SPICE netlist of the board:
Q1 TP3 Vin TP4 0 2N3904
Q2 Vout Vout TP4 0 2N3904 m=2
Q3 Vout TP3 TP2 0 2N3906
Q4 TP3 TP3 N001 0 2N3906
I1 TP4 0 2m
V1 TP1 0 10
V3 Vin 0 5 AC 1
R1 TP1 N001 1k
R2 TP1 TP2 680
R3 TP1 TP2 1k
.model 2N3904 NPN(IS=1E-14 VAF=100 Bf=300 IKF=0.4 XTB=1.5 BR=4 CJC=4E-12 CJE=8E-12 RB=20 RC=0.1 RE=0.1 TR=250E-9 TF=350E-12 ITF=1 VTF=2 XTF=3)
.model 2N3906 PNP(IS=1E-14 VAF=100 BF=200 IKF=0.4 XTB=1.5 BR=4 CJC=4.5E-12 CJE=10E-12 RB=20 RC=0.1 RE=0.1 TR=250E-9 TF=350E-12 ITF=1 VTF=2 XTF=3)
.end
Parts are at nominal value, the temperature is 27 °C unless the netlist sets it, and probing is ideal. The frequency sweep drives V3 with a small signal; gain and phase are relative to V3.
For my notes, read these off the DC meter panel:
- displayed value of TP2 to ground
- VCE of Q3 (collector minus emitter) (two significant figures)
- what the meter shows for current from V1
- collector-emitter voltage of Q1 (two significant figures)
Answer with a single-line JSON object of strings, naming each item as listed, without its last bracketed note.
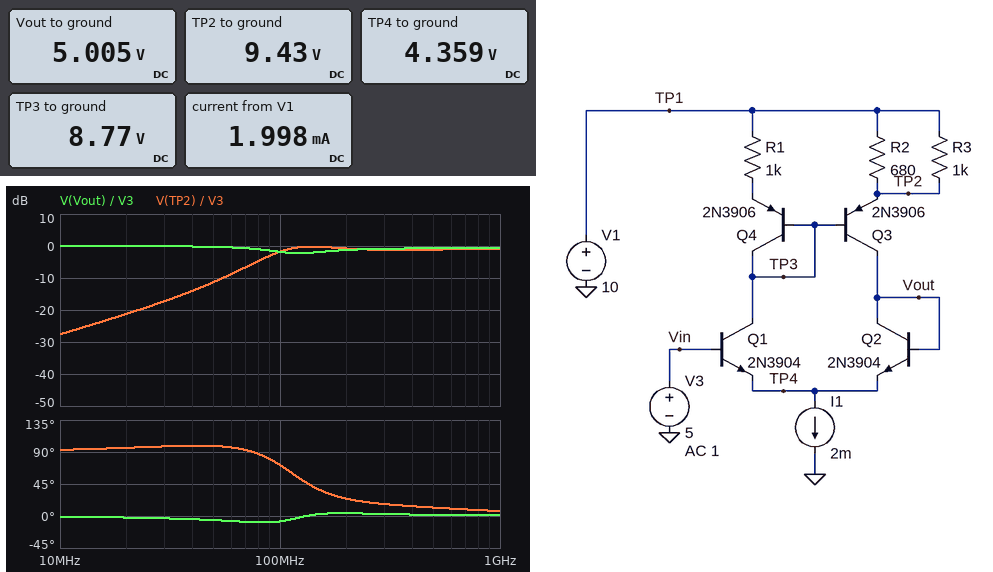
{"displayed value of TP2 to ground": "9.43 V", "VCE of Q3 (collector minus emitter)": "-4.4 V", "what the meter shows for current from V1": "1.998 mA", "collector-emitter voltage of Q1": "4.4 V"}
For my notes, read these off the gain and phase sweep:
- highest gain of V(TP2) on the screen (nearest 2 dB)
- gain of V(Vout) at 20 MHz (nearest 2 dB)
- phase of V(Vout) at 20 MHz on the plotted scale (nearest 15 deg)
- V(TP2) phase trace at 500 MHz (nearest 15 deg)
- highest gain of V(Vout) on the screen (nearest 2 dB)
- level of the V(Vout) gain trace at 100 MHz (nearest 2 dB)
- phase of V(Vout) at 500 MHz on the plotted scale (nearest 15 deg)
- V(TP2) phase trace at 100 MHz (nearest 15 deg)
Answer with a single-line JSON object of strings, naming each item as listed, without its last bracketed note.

{"highest gain of V(TP2) on the screen": "0 dB", "gain of V(Vout) at 20 MHz": "0 dB", "phase of V(Vout) at 20 MHz on the plotted scale": "0 deg", "V(TP2) phase trace at 500 MHz": "15 deg", "highest gain of V(Vout) on the screen": "0 dB", "level of the V(Vout) gain trace at 100 MHz": "-2 dB", "phase of V(Vout) at 500 MHz on the plotted scale": "0 deg", "V(TP2) phase trace at 100 MHz": "75 deg"}
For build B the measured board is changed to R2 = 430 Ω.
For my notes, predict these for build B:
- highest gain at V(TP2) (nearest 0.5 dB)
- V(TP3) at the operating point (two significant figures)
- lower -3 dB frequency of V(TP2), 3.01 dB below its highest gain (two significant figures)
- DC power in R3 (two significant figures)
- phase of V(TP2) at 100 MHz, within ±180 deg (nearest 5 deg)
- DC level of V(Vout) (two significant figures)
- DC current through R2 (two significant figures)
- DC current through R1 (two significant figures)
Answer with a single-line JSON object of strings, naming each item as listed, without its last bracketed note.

{"highest gain at V(TP2)": "-0.5 dB", "V(TP3) at the operating point": "8.9 V", "lower -3 dB frequency of V(TP2), 3.01 dB below its highest gain": "91 MHz", "DC power in R3": "210 µW", "phase of V(TP2) at 100 MHz, within ±180 deg": "80 deg", "DC level of V(Vout)": "5.0 V", "DC current through R2": "1.1 mA", "DC current through R1": "480 µA"}
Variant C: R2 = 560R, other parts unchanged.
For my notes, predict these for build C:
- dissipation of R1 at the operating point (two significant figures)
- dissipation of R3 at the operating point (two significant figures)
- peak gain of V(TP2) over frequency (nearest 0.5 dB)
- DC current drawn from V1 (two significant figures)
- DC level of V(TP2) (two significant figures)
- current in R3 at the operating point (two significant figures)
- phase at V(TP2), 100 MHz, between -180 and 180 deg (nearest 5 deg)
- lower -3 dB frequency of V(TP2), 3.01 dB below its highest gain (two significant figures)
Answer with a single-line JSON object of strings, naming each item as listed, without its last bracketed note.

{"dissipation of R1 at the operating point": "300 µW", "dissipation of R3 at the operating point": "270 µW", "peak gain of V(TP2) over frequency": "-0.5 dB", "DC current drawn from V1": "2.0 mA", "DC level of V(TP2)": "9.5 V", "current in R3 at the operating point": "520 µA", "phase at V(TP2), 100 MHz, between -180 and 180 deg": "75 deg", "lower -3 dB frequency of V(TP2), 3.01 dB below its highest gain": "90 MHz"}
